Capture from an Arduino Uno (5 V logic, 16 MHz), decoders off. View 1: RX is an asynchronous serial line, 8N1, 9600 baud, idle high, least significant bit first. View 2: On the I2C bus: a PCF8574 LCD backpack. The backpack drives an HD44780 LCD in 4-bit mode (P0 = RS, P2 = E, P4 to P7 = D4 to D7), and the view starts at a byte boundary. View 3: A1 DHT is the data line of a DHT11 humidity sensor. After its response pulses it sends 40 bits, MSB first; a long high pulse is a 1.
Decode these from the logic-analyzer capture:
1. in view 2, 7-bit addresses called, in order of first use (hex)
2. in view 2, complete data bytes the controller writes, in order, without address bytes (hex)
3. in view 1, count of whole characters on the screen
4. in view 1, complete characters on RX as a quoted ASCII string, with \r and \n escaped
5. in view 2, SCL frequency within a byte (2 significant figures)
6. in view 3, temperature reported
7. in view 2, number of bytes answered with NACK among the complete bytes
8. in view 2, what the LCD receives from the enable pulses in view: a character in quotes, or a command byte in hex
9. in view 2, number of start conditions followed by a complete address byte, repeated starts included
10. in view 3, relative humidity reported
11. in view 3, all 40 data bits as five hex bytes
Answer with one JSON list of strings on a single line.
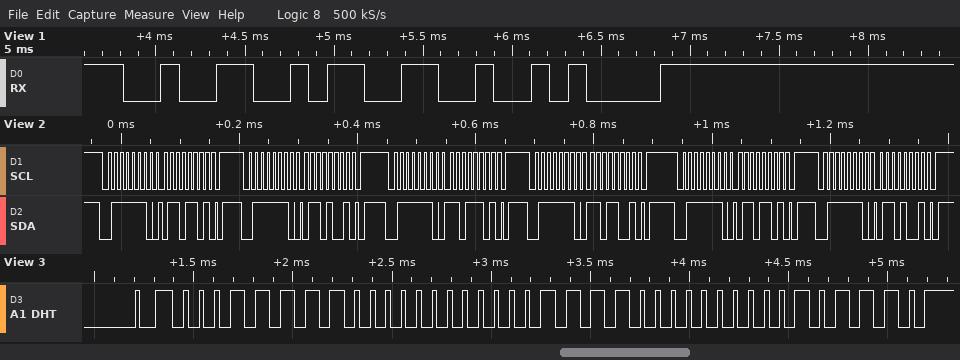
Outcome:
["0x3F", "6D 69 DD D9 6D 69", "3", "\"23\\n\"", "100 kHz", "15.0 °C", "0", "'m'", "6", "31 %", "1F 00 0F 00 2E"]
